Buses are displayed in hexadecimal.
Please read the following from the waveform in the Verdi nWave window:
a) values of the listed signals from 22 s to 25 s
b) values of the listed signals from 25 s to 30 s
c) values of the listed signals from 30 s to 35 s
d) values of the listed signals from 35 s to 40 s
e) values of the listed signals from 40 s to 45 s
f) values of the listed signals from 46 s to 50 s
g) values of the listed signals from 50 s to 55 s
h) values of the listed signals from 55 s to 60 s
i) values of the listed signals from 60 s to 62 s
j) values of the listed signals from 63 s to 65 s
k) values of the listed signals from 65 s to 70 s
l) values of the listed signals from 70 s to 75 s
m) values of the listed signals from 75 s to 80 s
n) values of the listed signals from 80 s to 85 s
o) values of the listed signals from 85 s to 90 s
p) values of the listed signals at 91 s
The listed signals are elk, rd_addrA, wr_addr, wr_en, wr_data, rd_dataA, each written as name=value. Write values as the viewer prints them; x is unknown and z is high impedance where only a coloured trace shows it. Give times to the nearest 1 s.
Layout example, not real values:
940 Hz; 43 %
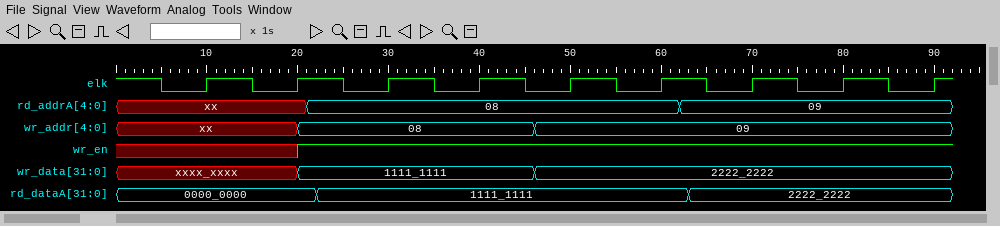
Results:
elk=1, rd_addrA=08, wr_addr=08, wr_en=1, wr_data=1111_1111, rd_dataA=1111_1111; elk=0, rd_addrA=08, wr_addr=08, wr_en=1, wr_data=1111_1111, rd_dataA=1111_1111; elk=1, rd_addrA=08, wr_addr=08, wr_en=1, wr_data=1111_1111, rd_dataA=1111_1111; elk=0, rd_addrA=08, wr_addr=08, wr_en=1, wr_data=1111_1111, rd_dataA=1111_1111; elk=1, rd_addrA=08, wr_addr=08, wr_en=1, wr_data=1111_1111, rd_dataA=1111_1111; elk=0, rd_addrA=08, wr_addr=09, wr_en=1, wr_data=2222_2222, rd_dataA=1111_1111; elk=1, rd_addrA=08, wr_addr=09, wr_en=1, wr_data=2222_2222, rd_dataA=1111_1111; elk=0, rd_addrA=08, wr_addr=09, wr_en=1, wr_data=2222_2222, rd_dataA=1111_1111; elk=1, rd_addrA=08, wr_addr=09, wr_en=1, wr_data=2222_2222, rd_dataA=1111_1111; elk=1, rd_addrA=09, wr_addr=09, wr_en=1, wr_data=2222_2222, rd_dataA=2222_2222; elk=0, rd_addrA=09, wr_addr=09, wr_en=1, wr_data=2222_2222, rd_dataA=2222_2222; elk=1, rd_addrA=09, wr_addr=09, wr_en=1, wr_data=2222_2222, rd_dataA=2222_2222; elk=0, rd_addrA=09, wr_addr=09, wr_en=1, wr_data=2222_2222, rd_dataA=2222_2222; elk=1, rd_addrA=09, wr_addr=09, wr_en=1, wr_data=2222_2222, rd_dataA=2222_2222; elk=0, rd_addrA=09, wr_addr=09, wr_en=1, wr_data=2222_2222, rd_dataA=2222_2222; elk=1, rd_addrA=09, wr_addr=09, wr_en=1, wr_data=2222_2222, rd_dataA=2222_2222
